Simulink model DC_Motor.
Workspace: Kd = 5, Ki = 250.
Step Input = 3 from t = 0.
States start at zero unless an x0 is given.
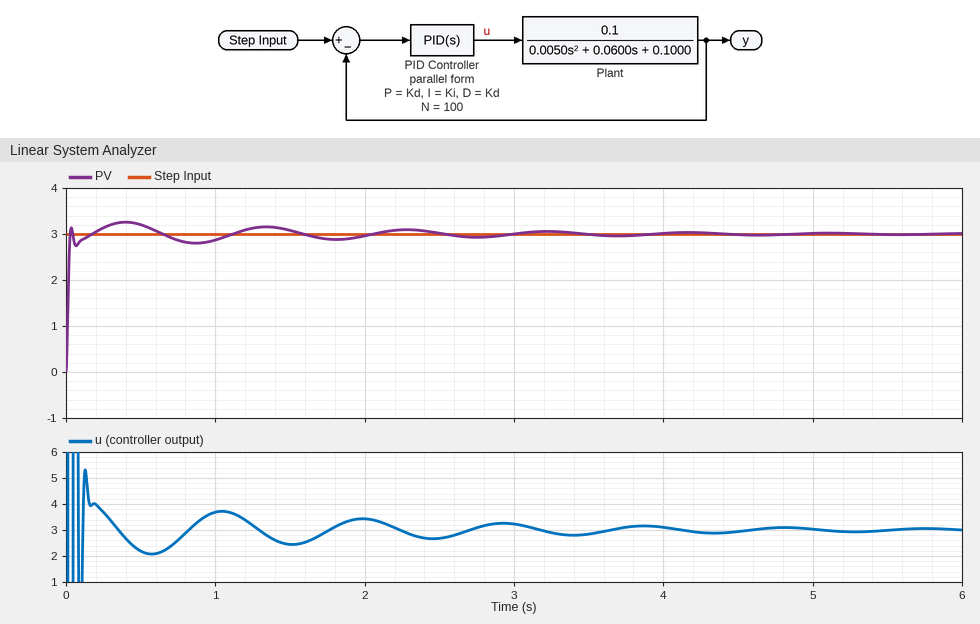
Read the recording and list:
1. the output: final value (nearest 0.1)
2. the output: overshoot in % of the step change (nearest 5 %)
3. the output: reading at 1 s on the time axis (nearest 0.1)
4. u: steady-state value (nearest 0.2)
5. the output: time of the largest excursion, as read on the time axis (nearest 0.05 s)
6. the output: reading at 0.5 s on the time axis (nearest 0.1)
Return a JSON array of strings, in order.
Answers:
["3.0", "10 %", "2.9", "3.0", "0.40 s", "3.2"]
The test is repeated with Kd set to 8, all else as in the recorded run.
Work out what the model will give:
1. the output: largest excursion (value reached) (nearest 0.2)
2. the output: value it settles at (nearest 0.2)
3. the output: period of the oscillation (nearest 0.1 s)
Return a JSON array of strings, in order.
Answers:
["3.4", "3.0", "0.5 s"]
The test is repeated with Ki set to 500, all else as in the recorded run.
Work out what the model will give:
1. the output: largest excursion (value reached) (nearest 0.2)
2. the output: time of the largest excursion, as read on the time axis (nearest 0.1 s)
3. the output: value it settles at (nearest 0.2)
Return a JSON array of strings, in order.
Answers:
["3.4", "0.3 s", "3.0"]
